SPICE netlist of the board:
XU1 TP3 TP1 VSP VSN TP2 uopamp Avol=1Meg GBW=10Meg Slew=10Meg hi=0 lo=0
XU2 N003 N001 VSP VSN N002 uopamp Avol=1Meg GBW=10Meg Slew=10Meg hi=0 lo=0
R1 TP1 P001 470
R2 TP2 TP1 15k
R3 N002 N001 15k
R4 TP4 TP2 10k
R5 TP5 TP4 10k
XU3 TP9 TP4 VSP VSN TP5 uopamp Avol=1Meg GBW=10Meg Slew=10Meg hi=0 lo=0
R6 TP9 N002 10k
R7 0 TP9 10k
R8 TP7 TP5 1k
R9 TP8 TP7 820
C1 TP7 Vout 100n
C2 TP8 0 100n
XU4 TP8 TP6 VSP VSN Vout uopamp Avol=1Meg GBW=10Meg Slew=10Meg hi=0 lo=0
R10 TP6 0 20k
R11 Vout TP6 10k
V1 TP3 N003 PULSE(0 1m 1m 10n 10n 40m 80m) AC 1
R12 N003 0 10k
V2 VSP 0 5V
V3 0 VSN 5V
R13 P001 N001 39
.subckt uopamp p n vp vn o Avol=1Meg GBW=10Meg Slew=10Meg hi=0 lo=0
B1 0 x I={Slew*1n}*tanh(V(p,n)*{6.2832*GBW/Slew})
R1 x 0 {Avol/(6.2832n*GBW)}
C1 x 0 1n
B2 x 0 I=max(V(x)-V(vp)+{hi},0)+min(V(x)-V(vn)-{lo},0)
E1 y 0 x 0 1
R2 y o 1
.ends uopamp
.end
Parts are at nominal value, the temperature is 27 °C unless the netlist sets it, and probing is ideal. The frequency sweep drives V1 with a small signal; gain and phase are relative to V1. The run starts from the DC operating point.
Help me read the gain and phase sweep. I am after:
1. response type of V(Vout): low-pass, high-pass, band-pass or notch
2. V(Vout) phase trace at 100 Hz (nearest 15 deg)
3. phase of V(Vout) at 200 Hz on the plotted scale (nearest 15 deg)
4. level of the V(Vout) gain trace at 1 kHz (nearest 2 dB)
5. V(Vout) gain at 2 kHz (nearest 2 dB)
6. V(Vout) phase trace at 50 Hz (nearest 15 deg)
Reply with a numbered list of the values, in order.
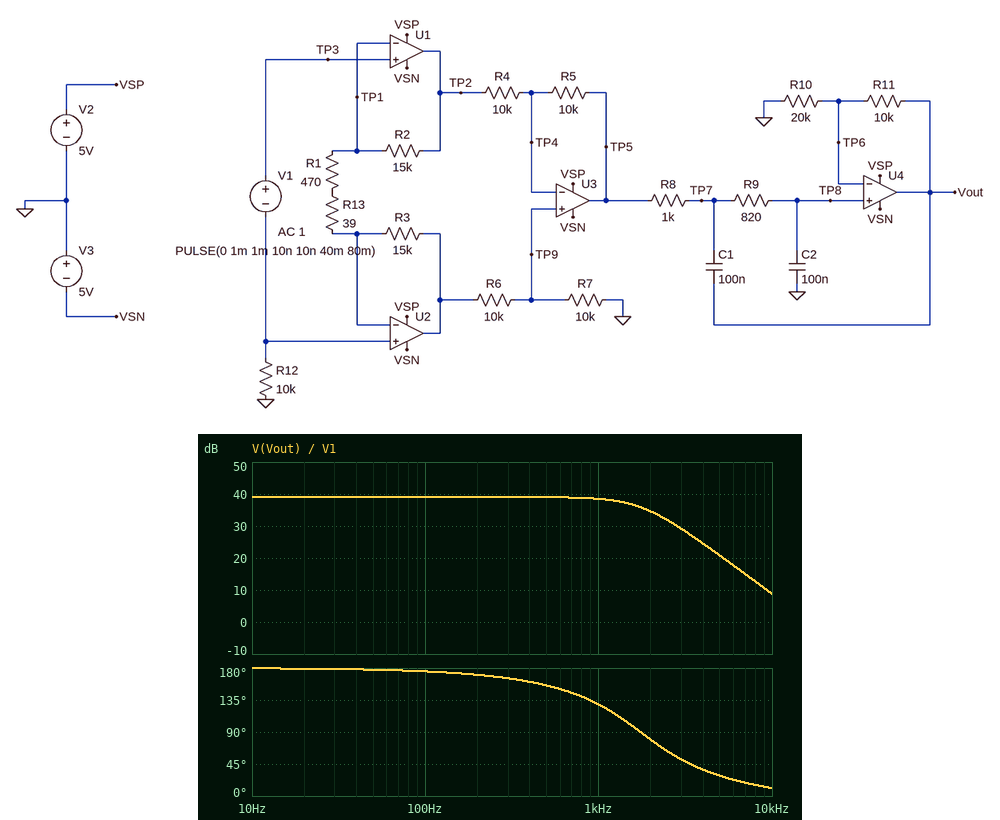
1. low-pass
2. 180 deg
3. 165 deg
4. 38 dB
5. 34 dB
6. 180 deg
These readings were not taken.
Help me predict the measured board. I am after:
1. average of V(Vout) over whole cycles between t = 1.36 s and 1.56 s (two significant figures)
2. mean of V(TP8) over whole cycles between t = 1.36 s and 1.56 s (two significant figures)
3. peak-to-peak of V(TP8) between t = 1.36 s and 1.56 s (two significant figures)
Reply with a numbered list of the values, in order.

1. -45 mV
2. -30 mV
3. 65 mV
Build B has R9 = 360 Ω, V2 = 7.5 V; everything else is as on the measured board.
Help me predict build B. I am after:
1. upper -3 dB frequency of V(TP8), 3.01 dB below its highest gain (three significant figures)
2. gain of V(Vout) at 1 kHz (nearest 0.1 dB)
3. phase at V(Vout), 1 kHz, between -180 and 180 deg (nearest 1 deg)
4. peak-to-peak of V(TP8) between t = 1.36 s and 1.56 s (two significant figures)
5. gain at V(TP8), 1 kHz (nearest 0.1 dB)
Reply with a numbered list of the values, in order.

1. 2.62 kHz
2. 39.0 dB
3. 147 deg
4. 66 mV
5. 35.4 dB
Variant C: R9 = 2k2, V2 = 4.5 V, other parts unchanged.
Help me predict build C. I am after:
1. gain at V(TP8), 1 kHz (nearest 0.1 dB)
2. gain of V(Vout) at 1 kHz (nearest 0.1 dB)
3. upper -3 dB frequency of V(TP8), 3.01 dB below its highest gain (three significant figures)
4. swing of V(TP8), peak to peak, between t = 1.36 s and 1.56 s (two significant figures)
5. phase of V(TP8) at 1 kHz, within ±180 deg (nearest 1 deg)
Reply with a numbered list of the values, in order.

1. 30.9 dB
2. 34.5 dB
3. 788 Hz
4. 60 mV
5. 94 deg
